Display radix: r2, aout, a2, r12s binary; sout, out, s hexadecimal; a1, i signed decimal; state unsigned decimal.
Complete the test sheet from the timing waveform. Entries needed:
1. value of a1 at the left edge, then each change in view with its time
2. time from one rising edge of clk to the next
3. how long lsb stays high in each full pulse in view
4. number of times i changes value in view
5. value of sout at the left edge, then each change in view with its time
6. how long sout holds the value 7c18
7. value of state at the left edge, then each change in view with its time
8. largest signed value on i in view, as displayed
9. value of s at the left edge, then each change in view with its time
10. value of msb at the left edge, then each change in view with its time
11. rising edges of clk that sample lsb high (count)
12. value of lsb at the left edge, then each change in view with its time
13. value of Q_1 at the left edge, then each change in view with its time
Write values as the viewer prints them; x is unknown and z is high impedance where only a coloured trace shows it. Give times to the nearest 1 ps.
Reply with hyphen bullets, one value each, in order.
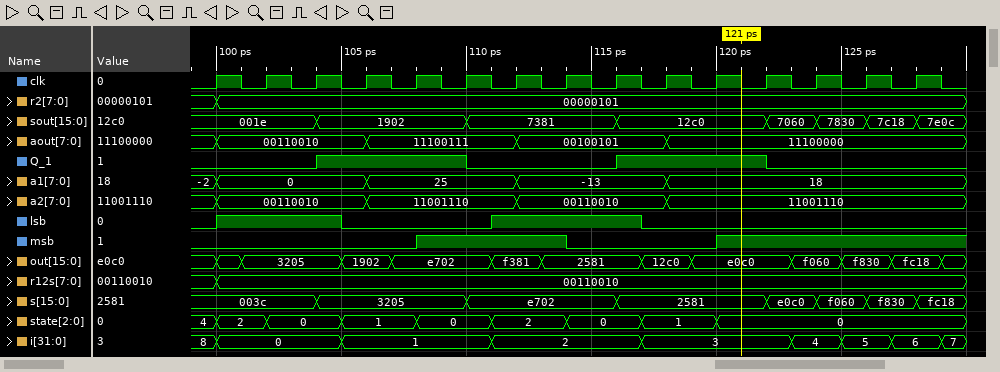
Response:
- -2, 0 at 100 ps, 25 at 106 ps, -13 at 112 ps, 18 at 118 ps
- 2 ps
- 5 ps, 6 ps
- 8
- 001e, 1902 at 104 ps, 7381 at 110 ps, 12c0 at 116 ps, 7060 at 122 ps, 7830 at 124 ps, 7c18 at 126 ps, 7e0c at 128 ps
- 2 ps
- 4, 2 at 100 ps, 0 at 102 ps, 1 at 105 ps, 0 at 108 ps, 2 at 111 ps, 0 at 114 ps, 1 at 117 ps, 0 at 120 ps
- 8
- 003c, 3205 at 104 ps, e702 at 110 ps, 2581 at 116 ps, e0c0 at 122 ps, f060 at 124 ps, f830 at 126 ps, fc18 at 128 ps
- 0, 1 at 108 ps, 0 at 114 ps, 1 at 120 ps
- 5
- 0, 1 at 100 ps, 0 at 105 ps, 1 at 111 ps, 0 at 117 ps
- 0, 1 at 104 ps, 0 at 110 ps, 1 at 116 ps, 0 at 122 ps
